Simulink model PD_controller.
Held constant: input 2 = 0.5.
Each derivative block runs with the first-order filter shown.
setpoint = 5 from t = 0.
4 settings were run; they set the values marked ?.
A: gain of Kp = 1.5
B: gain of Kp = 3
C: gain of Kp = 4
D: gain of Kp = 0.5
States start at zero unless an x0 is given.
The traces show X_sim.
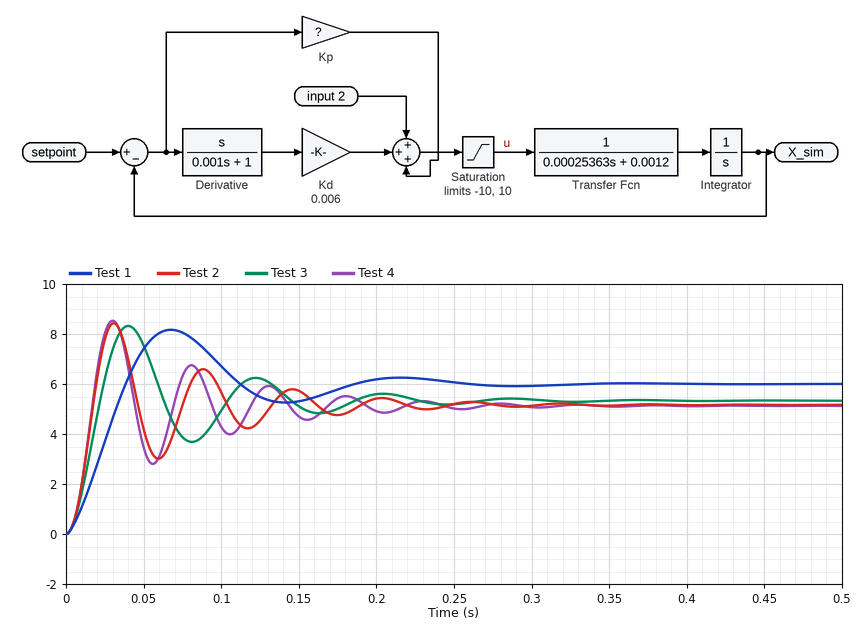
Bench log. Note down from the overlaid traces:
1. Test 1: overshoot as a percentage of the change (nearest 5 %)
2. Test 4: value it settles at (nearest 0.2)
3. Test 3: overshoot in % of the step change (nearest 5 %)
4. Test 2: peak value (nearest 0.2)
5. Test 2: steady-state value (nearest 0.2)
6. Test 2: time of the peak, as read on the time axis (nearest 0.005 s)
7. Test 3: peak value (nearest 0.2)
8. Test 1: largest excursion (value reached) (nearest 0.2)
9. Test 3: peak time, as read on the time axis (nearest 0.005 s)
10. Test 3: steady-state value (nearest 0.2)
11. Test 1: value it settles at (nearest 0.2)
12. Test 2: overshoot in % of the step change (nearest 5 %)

35 %
5.2
55 %
8.4
5.2
0.030 s
8.4
8.2
0.040 s
5.4
6.0
65 %
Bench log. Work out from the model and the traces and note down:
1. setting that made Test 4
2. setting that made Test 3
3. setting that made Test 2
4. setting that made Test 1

C
A
B
D
